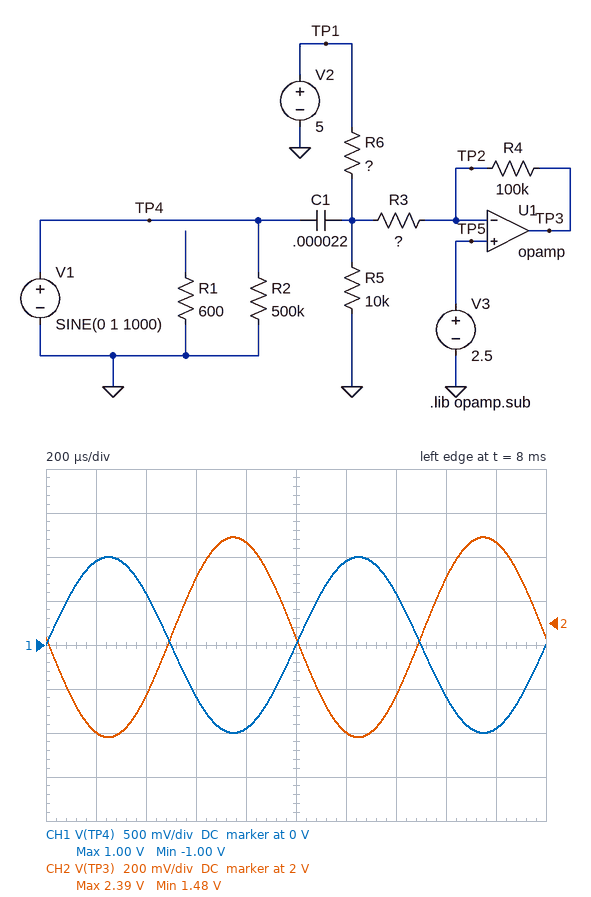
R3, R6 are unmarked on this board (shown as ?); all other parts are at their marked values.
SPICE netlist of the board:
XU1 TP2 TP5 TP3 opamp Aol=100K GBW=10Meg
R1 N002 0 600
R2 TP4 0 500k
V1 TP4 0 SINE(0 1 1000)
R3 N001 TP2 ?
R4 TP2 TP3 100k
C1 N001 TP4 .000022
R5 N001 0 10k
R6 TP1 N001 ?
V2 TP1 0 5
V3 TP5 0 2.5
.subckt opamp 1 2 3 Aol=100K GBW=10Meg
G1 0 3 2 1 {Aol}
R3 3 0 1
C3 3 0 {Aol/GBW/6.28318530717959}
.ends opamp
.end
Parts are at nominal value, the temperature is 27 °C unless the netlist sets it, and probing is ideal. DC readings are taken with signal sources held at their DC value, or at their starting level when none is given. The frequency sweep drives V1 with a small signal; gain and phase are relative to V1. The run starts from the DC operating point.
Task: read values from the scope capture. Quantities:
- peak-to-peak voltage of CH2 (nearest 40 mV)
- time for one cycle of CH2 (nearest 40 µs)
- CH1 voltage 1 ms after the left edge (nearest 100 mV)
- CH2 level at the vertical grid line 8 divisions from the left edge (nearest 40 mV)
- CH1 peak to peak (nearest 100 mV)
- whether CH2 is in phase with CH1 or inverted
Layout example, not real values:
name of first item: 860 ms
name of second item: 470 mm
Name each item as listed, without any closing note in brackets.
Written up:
peak-to-peak voltage of CH2: 920 mV
time for one cycle of CH2: 1.00 ms
CH1 voltage 1 ms after the left edge: 0 V
CH2 level at the vertical grid line 8 divisions from the left edge: 2.20 V
CH1 peak to peak: 2.0 V
whether CH2 is in phase with CH1 or inverted: inverted
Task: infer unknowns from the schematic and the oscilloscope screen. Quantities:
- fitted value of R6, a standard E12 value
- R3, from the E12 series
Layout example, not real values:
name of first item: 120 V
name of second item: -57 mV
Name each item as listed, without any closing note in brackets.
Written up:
fitted value of R6, a standard E12 value: 3.3 kΩ
R3, from the E12 series: 220 kΩ
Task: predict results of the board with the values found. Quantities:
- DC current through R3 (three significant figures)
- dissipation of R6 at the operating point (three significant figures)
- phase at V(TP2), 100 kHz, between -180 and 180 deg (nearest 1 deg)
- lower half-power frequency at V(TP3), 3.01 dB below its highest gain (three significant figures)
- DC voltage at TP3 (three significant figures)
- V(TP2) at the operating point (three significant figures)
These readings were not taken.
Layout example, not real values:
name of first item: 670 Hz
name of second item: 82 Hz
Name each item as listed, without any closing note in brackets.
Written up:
DC current through R3: 5.66 µA
dissipation of R6 at the operating point: 477 µW
phase at V(TP2), 100 kHz, between -180 and 180 deg: 89 deg
lower half-power frequency at V(TP3), 3.01 dB below its highest gain: 2.95 Hz
DC voltage at TP3: 1.93 V
V(TP2) at the operating point: 2.50 V
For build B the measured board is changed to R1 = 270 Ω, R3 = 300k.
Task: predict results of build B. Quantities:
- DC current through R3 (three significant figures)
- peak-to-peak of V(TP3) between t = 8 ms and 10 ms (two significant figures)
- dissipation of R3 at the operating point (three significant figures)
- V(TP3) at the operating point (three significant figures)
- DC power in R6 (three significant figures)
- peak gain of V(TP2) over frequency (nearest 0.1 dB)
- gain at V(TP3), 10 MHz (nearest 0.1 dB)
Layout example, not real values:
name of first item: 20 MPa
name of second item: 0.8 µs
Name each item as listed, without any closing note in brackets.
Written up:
DC current through R3: 4.16 µA
peak-to-peak of V(TP3) between t = 8 ms and 10 ms: 670 mV
dissipation of R3 at the operating point: 5.20 µW
V(TP3) at the operating point: 2.08 V
DC power in R6: 474 µW
peak gain of V(TP2) over frequency: -12.0 dB
gain at V(TP3), 10 MHz: -14.0 dB
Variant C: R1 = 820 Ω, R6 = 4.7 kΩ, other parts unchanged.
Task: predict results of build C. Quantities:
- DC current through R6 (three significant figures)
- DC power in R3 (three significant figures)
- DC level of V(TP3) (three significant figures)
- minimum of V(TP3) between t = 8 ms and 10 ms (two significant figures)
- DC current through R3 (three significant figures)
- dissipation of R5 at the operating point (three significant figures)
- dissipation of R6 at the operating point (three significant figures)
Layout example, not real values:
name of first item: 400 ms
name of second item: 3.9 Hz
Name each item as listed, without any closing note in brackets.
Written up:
DC current through R6: 343 µA
DC power in R3: 3.59 µW
DC level of V(TP3): 2.10 V
minimum of V(TP3) between t = 8 ms and 10 ms: 1.6 V
DC current through R3: 4.04 µA
dissipation of R5 at the operating point: 1.15 mW
dissipation of R6 at the operating point: 553 µW
